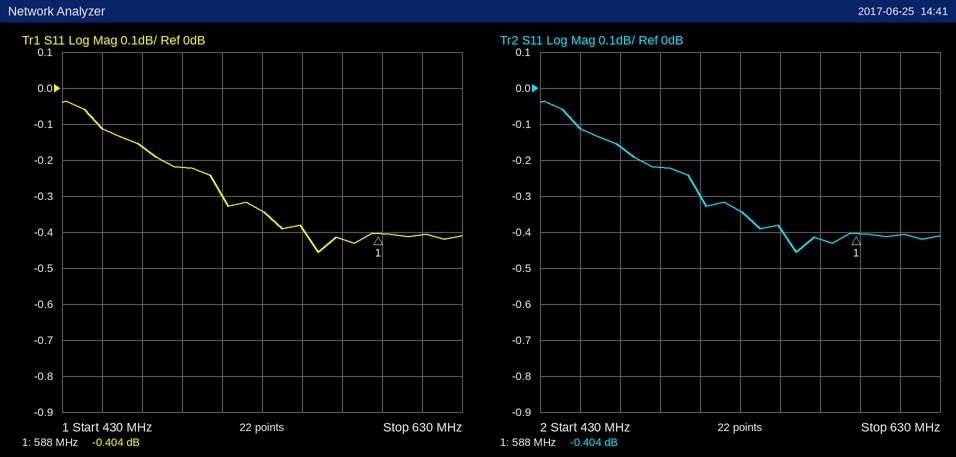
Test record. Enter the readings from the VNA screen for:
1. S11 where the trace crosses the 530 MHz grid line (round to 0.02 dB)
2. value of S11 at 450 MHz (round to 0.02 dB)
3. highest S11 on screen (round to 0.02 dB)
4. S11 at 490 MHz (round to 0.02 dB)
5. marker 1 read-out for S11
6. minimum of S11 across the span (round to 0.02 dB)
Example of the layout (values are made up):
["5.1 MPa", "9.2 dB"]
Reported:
["-0.34 dB", "-0.12 dB", "-0.04 dB", "-0.22 dB", "-0.404 dB", "-0.46 dB"]
